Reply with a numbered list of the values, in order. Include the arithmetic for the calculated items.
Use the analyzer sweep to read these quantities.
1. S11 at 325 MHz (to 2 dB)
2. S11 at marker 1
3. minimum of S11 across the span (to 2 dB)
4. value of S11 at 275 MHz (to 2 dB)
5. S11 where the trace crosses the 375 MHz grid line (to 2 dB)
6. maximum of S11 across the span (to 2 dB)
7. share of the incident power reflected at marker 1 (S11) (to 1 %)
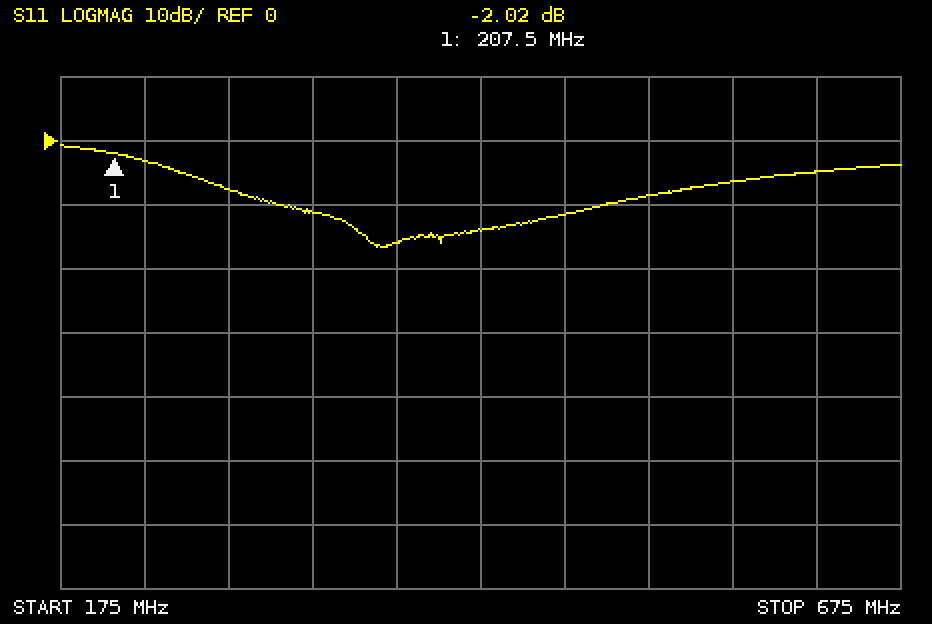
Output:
1. -12 dB
2. -2.02 dB
3. -16 dB
4. -8 dB
5. -16 dB
6. 0 dB
7. 10^(-2.02/10) ≈ 63 %
